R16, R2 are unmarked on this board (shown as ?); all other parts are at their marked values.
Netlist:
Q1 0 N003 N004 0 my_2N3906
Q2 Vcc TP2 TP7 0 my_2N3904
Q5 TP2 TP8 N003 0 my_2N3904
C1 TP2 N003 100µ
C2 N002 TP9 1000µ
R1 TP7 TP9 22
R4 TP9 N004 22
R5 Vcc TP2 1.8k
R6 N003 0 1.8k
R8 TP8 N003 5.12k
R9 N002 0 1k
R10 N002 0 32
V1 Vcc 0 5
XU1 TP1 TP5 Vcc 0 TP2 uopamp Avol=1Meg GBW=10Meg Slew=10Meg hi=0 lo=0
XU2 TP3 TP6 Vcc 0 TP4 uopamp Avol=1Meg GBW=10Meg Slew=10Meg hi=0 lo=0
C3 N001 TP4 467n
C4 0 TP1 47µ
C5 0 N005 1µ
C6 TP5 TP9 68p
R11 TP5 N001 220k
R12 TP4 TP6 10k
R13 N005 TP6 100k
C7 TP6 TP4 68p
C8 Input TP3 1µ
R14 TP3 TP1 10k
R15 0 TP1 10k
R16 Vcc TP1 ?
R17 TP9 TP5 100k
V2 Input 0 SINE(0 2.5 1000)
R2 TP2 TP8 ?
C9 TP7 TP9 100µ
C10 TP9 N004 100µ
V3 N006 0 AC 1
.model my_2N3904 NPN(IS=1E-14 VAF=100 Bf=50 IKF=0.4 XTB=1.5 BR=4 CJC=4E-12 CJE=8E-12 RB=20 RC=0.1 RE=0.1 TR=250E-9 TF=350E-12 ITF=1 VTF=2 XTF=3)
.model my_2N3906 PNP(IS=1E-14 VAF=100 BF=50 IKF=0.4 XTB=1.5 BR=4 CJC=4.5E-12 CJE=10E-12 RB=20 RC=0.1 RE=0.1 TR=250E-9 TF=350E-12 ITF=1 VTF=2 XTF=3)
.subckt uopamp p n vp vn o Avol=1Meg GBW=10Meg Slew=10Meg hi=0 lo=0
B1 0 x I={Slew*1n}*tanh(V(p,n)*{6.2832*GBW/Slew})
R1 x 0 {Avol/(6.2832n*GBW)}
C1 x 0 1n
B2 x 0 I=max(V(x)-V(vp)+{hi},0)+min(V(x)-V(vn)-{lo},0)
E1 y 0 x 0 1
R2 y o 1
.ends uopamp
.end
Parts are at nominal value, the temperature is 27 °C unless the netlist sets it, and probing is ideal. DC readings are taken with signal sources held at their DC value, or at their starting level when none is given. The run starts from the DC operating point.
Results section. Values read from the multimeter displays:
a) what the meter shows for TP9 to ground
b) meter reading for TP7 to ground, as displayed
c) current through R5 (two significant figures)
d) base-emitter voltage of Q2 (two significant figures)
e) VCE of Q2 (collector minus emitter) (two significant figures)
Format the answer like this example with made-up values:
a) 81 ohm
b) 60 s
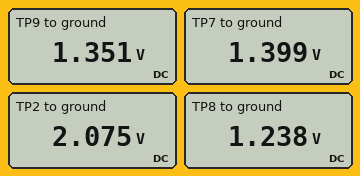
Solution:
a) 1.351 V
b) 1.399 V
c) 1.6 mA
d) 680 mV
e) 3.6 V
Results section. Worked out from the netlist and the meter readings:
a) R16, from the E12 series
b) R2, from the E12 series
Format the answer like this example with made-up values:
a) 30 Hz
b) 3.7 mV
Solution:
a) 27 kΩ
b) 6.8 kΩ
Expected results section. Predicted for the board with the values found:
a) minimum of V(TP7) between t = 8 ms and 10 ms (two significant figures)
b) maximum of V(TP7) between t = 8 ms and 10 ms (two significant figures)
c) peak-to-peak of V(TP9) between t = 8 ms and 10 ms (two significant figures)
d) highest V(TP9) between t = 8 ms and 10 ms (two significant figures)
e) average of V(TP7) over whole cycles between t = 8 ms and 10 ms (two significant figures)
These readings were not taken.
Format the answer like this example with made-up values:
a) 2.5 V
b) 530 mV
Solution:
a) 450 mV
b) 2.2 V
c) 1.7 V
d) 2.0 V
e) 1.4 V
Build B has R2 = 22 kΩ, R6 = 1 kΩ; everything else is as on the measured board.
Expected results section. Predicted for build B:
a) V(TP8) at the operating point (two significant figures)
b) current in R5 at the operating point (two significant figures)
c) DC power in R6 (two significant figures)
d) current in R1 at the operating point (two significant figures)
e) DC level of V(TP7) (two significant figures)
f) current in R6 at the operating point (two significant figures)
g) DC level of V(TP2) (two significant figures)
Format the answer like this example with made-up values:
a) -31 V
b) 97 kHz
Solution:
a) 720 mV
b) 1.5 mA
c) 110 µW
d) 13 mA
e) 1.6 V
f) 340 µA
g) 2.4 V
